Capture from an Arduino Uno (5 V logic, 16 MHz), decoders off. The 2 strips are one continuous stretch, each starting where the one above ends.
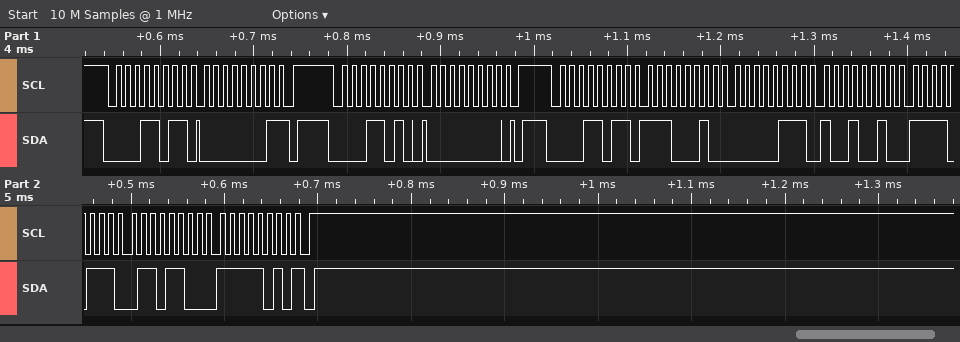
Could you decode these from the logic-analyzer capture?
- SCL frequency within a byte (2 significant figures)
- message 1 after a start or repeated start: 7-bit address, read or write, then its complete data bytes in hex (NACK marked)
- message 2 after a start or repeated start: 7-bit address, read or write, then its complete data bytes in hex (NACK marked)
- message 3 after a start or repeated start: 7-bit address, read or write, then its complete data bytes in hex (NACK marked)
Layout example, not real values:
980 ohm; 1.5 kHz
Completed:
100 kHz; 0x0D read: 01 NACK; 0x0D write: 00; 0x0D read: E2 07 92 F7 6C FA NACK
